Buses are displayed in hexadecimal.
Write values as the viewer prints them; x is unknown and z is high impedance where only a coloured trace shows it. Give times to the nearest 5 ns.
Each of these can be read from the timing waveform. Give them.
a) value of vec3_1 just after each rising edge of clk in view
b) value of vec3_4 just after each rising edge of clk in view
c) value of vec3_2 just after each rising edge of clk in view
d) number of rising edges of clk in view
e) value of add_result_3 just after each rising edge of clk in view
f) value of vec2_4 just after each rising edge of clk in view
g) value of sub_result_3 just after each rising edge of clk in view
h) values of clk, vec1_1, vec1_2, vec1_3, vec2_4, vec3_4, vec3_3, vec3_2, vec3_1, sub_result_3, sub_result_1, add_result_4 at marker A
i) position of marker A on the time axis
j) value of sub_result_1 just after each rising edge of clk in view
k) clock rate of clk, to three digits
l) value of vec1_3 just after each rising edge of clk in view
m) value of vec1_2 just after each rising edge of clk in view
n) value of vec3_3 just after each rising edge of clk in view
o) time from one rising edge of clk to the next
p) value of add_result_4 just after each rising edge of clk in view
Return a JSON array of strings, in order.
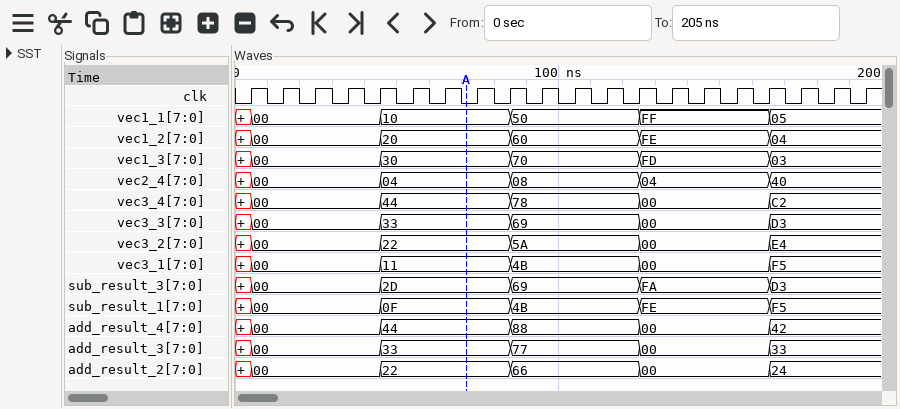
["00, 00, 00, 00, 11, 11, 11, 11, 4B, 4B, 4B, 4B, 00, 00, 00, 00, F5, F5, F5, F5", "00, 00, 00, 00, 44, 44, 44, 44, 78, 78, 78, 78, 00, 00, 00, 00, C2, C2, C2, C2", "00, 00, 00, 00, 22, 22, 22, 22, 5A, 5A, 5A, 5A, 00, 00, 00, 00, E4, E4, E4, E4", "20", "00, 00, 00, 00, 33, 33, 33, 33, 77, 77, 77, 77, 00, 00, 00, 00, 33, 33, 33, 33", "00, 00, 00, 00, 04, 04, 04, 04, 08, 08, 08, 08, 04, 04, 04, 04, 40, 40, 40, 40", "00, 00, 00, 00, 2D, 2D, 2D, 2D, 69, 69, 69, 69, FA, FA, FA, FA, D3, D3, D3, D3", "clk=0, vec1_1=10, vec1_2=20, vec1_3=30, vec2_4=04, vec3_4=44, vec3_3=33, vec3_2=22, vec3_1=11, sub_result_3=2D, sub_result_1=0F, add_result_4=44", "70 ns", "00, 00, 00, 00, 0F, 0F, 0F, 0F, 4B, 4B, 4B, 4B, FE, FE, FE, FE, F5, F5, F5, F5", "100 MHz", "00, 00, 00, 00, 30, 30, 30, 30, 70, 70, 70, 70, FD, FD, FD, FD, 03, 03, 03, 03", "00, 00, 00, 00, 20, 20, 20, 20, 60, 60, 60, 60, FE, FE, FE, FE, 04, 04, 04, 04", "00, 00, 00, 00, 33, 33, 33, 33, 69, 69, 69, 69, 00, 00, 00, 00, D3, D3, D3, D3", "10 ns", "00, 00, 00, 00, 44, 44, 44, 44, 88, 88, 88, 88, 00, 00, 00, 00, 42, 42, 42, 42"]
